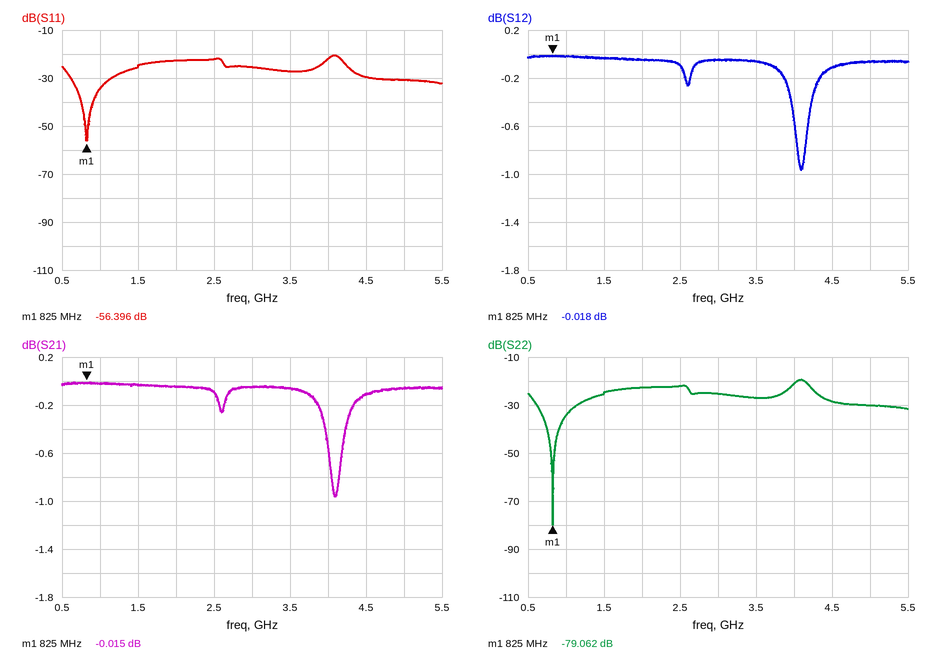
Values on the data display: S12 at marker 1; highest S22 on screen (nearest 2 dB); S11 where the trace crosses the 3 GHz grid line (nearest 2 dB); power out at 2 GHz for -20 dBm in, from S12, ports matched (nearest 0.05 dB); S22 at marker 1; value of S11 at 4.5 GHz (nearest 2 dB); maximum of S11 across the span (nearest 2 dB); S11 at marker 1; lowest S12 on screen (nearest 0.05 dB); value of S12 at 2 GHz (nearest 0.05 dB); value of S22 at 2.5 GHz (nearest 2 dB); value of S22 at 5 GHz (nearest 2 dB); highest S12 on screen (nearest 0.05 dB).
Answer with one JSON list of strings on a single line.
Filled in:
["-0.018 dB", "-20 dB", "-26 dB", "-20.05 dBm", "-79.062 dB", "-30 dB", "-20 dB", "-56.396 dB", "-0.95 dB", "-0.05 dB", "-22 dB", "-30 dB", "0.00 dB"]
